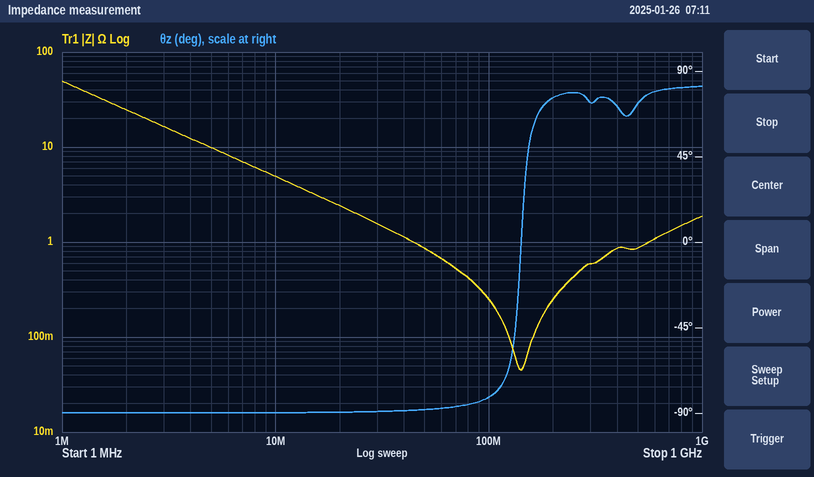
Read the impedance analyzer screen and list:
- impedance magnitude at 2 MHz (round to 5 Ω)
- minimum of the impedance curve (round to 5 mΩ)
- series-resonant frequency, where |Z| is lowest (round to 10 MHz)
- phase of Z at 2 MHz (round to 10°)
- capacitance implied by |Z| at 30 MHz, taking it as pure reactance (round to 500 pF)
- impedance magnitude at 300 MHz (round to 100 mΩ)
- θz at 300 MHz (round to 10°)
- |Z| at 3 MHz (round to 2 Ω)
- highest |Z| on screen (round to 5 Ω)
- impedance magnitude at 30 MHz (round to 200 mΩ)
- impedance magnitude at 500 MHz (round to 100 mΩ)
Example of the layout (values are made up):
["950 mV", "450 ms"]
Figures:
["25 Ω", "45 mΩ", "140 MHz", "-90°", "3.5 nF", "600 mΩ", "70°", "16 Ω", "50 Ω", "1.6 Ω", "900 mΩ"]
